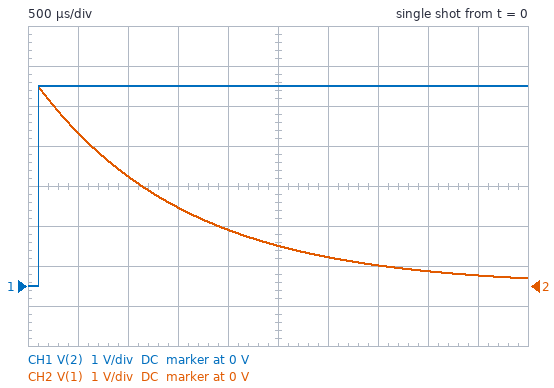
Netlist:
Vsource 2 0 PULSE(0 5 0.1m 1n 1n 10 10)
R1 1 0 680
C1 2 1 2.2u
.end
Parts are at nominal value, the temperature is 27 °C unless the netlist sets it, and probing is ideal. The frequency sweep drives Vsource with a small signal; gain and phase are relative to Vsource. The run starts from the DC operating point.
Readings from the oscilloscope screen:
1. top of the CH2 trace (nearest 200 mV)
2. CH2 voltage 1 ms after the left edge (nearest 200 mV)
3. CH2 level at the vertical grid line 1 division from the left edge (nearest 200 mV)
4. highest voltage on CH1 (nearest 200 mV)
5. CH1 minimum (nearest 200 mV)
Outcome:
5.0 V
2.8 V
3.8 V
5.0 V
0 V
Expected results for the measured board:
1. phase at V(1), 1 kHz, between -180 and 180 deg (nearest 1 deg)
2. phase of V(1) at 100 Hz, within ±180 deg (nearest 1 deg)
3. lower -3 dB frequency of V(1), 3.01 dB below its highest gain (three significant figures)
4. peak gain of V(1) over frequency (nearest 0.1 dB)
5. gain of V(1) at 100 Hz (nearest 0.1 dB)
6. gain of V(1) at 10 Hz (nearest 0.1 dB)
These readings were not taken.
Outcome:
6 deg
47 deg
106 Hz
0 dB
-3.3 dB
-20.6 dB
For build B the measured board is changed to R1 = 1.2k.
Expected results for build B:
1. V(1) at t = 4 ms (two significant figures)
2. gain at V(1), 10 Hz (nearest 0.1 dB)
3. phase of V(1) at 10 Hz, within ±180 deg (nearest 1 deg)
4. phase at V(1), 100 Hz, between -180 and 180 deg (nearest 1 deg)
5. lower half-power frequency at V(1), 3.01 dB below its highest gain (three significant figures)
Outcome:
1.1 V
-15.7 dB
81 deg
31 deg
60.3 Hz
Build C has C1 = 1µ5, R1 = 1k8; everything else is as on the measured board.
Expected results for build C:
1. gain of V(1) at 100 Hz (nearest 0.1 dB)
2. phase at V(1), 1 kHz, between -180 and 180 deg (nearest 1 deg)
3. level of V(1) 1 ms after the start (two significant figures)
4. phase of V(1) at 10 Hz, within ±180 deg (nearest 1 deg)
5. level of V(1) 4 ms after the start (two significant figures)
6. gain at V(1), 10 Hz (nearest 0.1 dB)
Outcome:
-1.3 dB
3 deg
3.6 V
80 deg
1.2 V
-15.5 dB
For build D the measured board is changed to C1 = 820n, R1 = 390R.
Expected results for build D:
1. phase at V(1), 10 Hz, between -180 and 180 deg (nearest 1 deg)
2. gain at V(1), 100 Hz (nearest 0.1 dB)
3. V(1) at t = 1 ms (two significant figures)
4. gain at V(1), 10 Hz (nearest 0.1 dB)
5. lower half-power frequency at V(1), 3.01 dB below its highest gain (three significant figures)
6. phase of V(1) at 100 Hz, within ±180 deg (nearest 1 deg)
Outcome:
89 deg
-14.1 dB
300 mV
-33.9 dB
498 Hz
79 deg
